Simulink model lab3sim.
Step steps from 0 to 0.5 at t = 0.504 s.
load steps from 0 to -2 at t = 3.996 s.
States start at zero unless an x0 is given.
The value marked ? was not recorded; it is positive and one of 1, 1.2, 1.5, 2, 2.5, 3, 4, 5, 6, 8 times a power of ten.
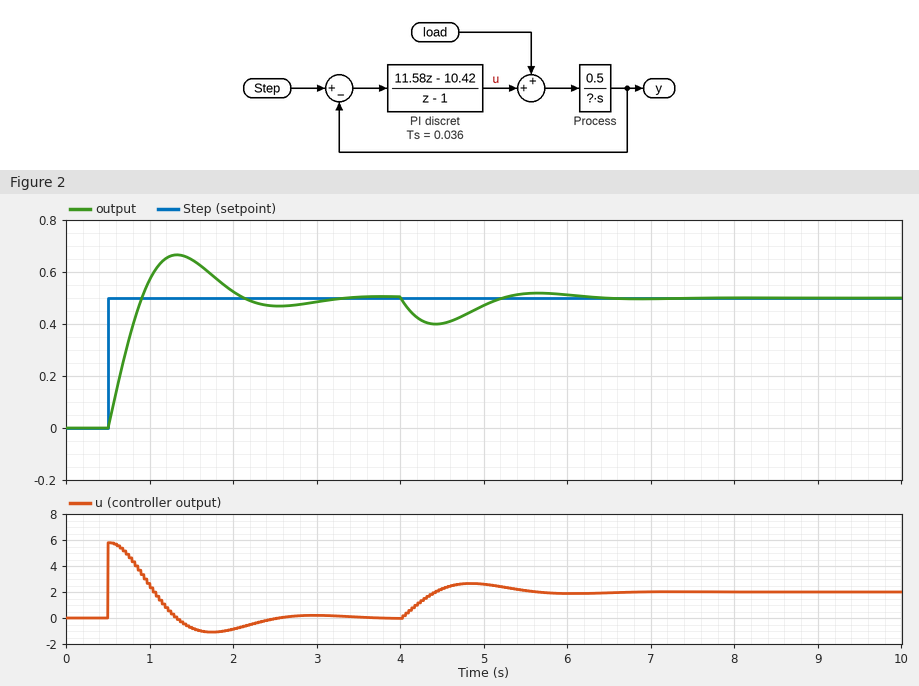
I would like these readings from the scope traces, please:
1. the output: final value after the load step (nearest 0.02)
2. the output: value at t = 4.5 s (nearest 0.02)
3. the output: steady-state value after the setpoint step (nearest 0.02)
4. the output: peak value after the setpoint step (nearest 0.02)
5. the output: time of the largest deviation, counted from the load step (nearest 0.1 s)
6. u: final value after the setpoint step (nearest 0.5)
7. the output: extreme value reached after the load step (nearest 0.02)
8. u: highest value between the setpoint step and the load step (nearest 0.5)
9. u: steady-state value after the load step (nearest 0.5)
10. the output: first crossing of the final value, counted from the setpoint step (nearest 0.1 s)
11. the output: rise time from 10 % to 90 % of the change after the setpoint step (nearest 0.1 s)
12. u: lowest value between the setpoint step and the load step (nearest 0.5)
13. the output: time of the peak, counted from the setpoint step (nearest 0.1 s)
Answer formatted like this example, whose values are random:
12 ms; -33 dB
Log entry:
0.50; 0.40; 0.50; 0.66; 0.4 s; 0.0; 0.40; 6.0; 2.0; 0.4 s; 0.3 s; -1.0; 0.8 s
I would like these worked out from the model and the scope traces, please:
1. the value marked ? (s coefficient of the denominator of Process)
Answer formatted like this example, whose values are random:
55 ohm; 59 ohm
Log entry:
2
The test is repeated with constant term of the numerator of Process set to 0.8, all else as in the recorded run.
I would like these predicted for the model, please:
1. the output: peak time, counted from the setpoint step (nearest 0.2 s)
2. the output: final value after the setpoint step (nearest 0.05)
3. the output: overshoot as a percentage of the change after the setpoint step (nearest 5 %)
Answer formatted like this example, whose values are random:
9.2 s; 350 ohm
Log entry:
0.6 s; 0.50; 25 %
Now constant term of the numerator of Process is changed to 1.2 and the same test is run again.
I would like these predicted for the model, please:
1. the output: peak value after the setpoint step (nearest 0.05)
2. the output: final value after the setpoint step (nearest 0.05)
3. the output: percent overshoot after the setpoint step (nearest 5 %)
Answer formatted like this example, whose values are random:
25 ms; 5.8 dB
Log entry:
0.60; 0.50; 20 %
